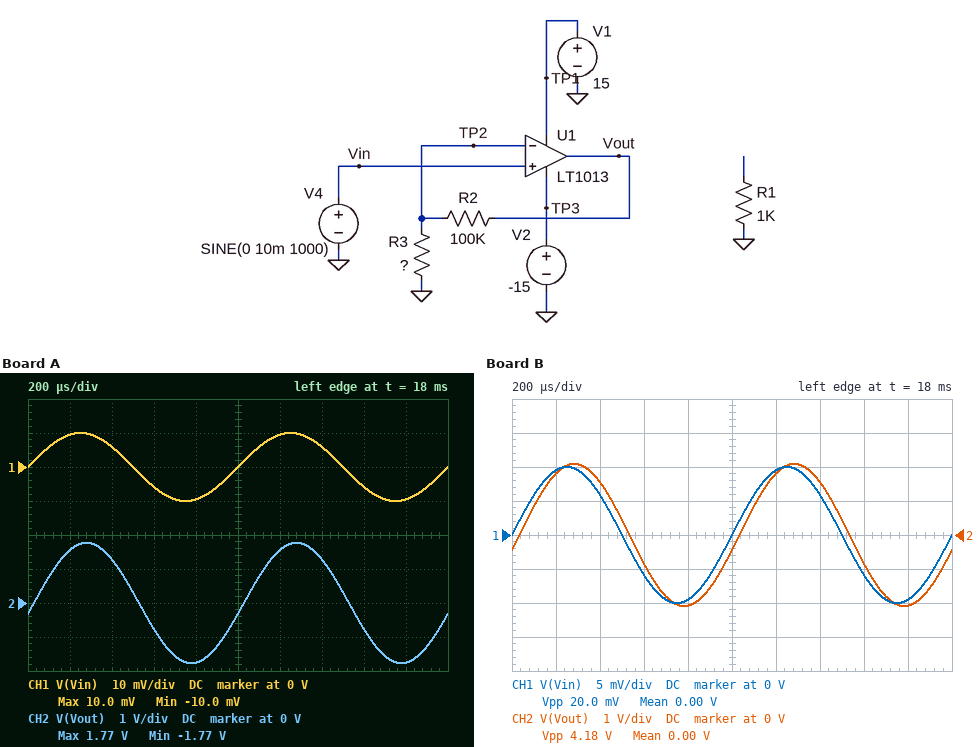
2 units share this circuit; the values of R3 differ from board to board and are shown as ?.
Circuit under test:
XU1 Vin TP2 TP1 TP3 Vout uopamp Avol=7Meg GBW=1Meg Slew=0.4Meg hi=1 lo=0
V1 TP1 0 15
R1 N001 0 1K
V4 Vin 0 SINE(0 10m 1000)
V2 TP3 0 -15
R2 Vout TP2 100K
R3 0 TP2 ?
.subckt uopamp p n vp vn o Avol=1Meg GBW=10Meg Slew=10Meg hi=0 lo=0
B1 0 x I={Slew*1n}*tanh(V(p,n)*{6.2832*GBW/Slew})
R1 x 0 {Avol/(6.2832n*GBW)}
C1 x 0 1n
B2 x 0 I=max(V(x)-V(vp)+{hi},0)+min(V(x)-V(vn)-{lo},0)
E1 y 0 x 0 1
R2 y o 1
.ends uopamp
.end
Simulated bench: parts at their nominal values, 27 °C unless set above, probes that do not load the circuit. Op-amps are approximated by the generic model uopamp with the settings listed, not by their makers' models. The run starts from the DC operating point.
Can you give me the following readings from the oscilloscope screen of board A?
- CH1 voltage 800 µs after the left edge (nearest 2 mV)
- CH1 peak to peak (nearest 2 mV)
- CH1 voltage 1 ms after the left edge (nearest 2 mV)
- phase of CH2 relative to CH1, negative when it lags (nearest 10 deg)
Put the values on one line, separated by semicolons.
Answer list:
-10 mV; 20 mV; 0 V; -10 deg
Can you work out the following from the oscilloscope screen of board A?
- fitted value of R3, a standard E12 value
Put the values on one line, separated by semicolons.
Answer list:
560 Ω
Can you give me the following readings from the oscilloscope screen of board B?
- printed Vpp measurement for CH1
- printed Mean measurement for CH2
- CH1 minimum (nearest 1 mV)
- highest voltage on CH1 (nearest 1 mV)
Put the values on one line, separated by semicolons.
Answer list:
20.0 mV; 0.00 V; -10 mV; 10 mV
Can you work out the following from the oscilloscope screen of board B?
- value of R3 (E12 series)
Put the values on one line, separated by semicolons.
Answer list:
470 Ω
